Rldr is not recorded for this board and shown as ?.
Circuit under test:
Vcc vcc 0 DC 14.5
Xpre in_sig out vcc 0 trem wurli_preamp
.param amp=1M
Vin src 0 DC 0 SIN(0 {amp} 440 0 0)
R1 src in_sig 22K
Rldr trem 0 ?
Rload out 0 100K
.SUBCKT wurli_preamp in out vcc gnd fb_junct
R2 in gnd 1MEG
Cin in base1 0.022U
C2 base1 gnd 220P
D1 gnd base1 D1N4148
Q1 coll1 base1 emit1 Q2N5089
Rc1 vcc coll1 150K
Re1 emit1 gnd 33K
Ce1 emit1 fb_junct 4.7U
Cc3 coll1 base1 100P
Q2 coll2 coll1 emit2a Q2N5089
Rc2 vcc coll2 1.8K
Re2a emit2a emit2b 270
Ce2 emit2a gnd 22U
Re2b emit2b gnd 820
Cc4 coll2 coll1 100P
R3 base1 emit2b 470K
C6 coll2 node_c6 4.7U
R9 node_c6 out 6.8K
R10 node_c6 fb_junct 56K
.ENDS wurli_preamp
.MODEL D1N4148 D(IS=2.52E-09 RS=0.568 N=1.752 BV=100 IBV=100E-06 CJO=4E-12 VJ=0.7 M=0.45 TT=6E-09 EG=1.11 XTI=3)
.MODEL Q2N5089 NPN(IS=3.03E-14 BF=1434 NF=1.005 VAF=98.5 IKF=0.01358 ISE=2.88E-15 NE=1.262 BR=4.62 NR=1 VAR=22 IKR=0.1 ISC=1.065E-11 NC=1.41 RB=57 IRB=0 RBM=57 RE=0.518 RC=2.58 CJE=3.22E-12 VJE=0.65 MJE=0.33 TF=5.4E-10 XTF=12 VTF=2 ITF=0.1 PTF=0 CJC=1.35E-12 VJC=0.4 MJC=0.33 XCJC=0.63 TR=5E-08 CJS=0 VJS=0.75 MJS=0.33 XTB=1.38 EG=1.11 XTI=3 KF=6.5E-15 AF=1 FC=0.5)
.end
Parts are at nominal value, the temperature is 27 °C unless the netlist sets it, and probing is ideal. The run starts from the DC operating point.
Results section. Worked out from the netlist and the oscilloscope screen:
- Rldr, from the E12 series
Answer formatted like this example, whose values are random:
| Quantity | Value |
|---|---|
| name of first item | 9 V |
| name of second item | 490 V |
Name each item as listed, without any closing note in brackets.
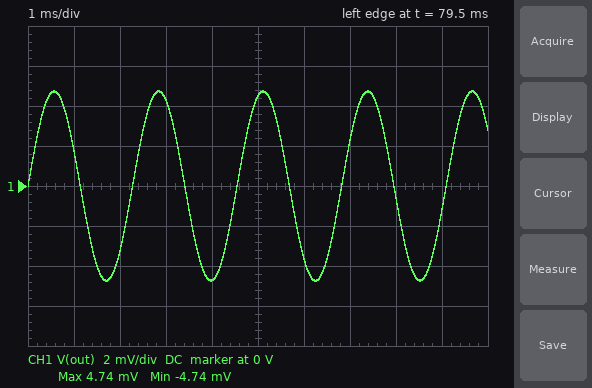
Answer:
| Quantity | Value |
|---|---|
| Rldr, from the E12 series | 18 kΩ |
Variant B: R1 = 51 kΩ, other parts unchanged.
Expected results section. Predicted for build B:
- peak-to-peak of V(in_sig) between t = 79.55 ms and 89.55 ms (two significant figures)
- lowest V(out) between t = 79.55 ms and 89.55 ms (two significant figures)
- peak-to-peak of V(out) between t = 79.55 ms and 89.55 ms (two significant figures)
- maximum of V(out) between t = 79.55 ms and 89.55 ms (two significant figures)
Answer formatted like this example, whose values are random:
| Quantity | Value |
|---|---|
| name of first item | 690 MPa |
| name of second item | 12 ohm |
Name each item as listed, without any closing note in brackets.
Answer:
| Quantity | Value |
|---|---|
| peak-to-peak of V(in_sig) between t = 79.55 ms and 89.55 ms | 1.7 mV |
| lowest V(out) between t = 79.55 ms and 89.55 ms | -4.4 mV |
| peak-to-peak of V(out) between t = 79.55 ms and 89.55 ms | 8.7 mV |
| maximum of V(out) between t = 79.55 ms and 89.55 ms | 4.4 mV |
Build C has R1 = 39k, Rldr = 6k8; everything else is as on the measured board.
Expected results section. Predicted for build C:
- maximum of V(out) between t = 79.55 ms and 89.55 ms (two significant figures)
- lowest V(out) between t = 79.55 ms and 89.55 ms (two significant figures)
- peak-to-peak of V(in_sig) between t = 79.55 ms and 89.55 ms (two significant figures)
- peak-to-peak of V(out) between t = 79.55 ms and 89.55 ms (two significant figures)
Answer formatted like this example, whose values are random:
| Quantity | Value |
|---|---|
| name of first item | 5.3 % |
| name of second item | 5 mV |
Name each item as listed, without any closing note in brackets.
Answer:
| Quantity | Value |
|---|---|
| maximum of V(out) between t = 79.55 ms and 89.55 ms | 8.5 mV |
| lowest V(out) between t = 79.55 ms and 89.55 ms | -8.5 mV |
| peak-to-peak of V(in_sig) between t = 79.55 ms and 89.55 ms | 1.8 mV |
| peak-to-peak of V(out) between t = 79.55 ms and 89.55 ms | 17 mV |
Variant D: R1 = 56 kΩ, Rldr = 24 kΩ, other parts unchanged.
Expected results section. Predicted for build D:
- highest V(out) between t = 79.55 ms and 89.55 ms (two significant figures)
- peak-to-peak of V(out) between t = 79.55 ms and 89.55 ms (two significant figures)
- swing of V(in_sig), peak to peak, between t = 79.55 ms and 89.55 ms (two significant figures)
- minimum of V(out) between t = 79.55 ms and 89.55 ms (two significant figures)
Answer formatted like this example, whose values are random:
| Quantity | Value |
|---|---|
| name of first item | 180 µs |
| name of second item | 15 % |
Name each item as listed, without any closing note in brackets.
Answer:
| Quantity | Value |
|---|---|
| highest V(out) between t = 79.55 ms and 89.55 ms | 3.7 mV |
| peak-to-peak of V(out) between t = 79.55 ms and 89.55 ms | 7.5 mV |
| swing of V(in_sig), peak to peak, between t = 79.55 ms and 89.55 ms | 1.7 mV |
| minimum of V(out) between t = 79.55 ms and 89.55 ms | -3.7 mV |
